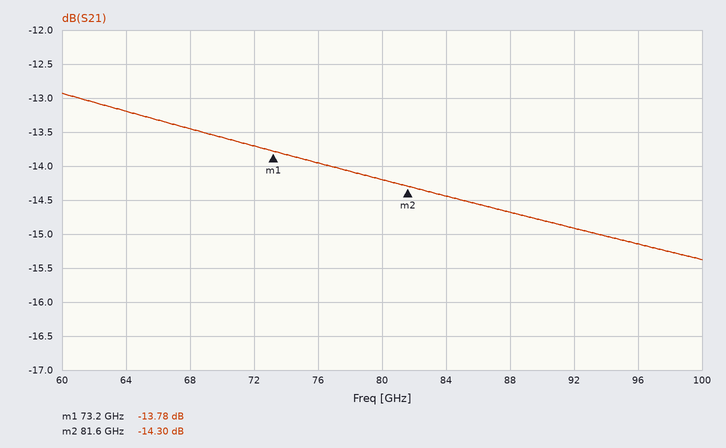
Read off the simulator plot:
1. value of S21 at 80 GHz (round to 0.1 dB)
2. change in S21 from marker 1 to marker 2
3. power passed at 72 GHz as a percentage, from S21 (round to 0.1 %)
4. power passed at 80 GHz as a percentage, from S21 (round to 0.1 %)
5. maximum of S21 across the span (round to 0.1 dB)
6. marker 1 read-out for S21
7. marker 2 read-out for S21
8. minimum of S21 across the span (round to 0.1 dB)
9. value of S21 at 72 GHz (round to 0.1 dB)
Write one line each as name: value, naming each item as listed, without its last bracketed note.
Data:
value of S21 at 80 GHz: -14.2 dB
change in S21 from marker 1 to marker 2: -0.52 dB
power passed at 72 GHz as a percentage, from S21: 4.3 %
power passed at 80 GHz as a percentage, from S21: 3.8 %
maximum of S21 across the span: -12.9 dB
marker 1 read-out for S21: -13.78 dB
marker 2 read-out for S21: -14.30 dB
minimum of S21 across the span: -15.4 dB
value of S21 at 72 GHz: -13.7 dB
